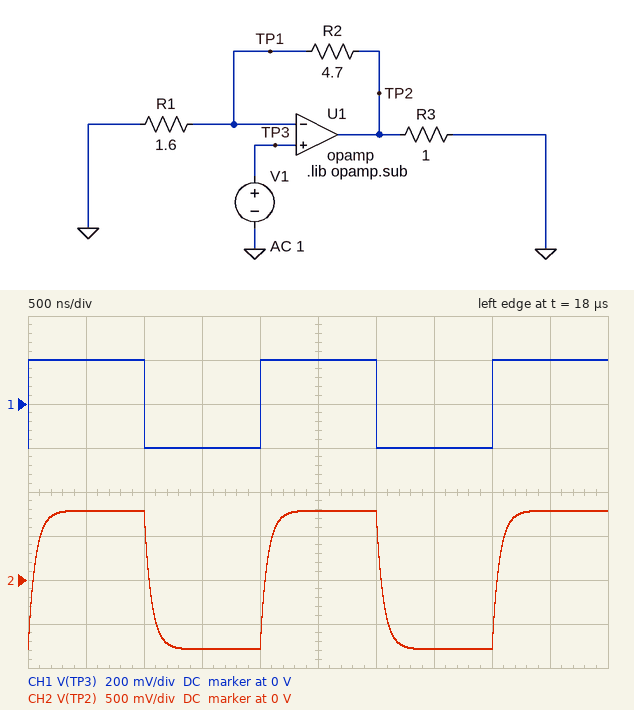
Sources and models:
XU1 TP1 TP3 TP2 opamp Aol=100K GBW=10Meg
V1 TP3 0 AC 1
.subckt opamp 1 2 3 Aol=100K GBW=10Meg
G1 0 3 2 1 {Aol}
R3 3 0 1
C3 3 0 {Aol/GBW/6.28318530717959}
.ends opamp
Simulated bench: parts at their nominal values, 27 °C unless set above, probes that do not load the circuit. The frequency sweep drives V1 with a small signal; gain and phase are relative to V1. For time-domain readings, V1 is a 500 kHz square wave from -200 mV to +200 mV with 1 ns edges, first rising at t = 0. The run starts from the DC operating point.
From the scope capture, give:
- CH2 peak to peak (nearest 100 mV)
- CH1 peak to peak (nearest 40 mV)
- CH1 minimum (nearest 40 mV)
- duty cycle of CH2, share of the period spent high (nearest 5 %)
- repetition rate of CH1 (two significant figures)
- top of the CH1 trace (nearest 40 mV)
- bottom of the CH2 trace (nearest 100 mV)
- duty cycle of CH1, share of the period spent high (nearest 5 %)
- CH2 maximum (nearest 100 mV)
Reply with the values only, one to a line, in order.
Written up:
1.6 V
400 mV
-200 mV
50 %
500 kHz
200 mV
-800 mV
50 %
800 mV
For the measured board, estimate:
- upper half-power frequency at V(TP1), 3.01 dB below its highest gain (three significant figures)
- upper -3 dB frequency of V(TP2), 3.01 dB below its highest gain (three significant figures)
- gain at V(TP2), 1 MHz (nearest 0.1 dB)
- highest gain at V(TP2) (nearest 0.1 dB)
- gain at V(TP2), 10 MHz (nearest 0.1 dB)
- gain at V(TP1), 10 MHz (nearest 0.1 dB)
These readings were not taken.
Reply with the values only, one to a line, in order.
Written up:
2.54 MHz
2.54 MHz
11.3 dB
11.9 dB
-0.3 dB
-12.2 dB
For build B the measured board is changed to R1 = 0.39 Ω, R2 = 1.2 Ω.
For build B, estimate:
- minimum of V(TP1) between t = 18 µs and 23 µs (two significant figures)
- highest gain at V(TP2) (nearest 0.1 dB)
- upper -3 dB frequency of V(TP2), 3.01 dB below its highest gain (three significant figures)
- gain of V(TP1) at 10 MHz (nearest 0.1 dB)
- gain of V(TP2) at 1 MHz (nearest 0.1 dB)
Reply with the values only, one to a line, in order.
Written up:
-200 mV
12.2 dB
2.45 MHz
-12.5 dB
11.5 dB
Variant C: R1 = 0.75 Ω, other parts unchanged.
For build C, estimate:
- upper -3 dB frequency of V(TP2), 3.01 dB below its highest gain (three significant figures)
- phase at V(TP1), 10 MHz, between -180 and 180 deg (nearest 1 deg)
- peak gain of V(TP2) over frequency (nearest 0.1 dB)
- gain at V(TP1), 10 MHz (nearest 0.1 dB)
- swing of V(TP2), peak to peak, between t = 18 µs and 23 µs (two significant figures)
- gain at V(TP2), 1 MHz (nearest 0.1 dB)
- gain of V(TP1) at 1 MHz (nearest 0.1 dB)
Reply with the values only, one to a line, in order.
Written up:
1.38 MHz
-82 deg
17.2 dB
-17.3 dB
2.9 V
15.4 dB
-1.8 dB
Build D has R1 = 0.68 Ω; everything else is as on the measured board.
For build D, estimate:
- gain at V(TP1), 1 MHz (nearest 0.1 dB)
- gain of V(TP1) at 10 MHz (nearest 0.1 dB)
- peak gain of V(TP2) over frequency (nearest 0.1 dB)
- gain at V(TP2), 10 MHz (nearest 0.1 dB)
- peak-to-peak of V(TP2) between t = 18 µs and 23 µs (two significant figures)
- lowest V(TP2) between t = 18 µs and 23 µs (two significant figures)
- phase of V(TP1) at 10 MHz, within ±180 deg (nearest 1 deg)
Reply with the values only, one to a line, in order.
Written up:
-2.1 dB
-18.0 dB
18.0 dB
-0.1 dB
3.2 V
-1.6 V
-83 deg
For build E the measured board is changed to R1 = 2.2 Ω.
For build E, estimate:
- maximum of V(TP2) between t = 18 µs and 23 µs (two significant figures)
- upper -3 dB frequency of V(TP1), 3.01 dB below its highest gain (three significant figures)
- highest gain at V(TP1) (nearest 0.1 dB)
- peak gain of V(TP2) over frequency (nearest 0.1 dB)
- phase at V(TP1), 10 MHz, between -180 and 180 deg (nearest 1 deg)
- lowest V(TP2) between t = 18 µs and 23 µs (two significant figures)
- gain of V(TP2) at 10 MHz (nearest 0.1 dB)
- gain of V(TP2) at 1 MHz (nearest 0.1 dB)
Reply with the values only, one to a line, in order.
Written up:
630 mV
3.19 MHz
0 dB
9.9 dB
-72 deg
-630 mV
-0.4 dB
9.5 dB
